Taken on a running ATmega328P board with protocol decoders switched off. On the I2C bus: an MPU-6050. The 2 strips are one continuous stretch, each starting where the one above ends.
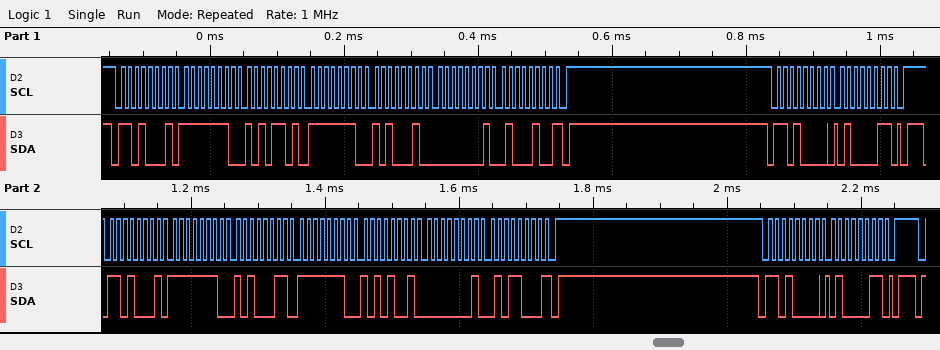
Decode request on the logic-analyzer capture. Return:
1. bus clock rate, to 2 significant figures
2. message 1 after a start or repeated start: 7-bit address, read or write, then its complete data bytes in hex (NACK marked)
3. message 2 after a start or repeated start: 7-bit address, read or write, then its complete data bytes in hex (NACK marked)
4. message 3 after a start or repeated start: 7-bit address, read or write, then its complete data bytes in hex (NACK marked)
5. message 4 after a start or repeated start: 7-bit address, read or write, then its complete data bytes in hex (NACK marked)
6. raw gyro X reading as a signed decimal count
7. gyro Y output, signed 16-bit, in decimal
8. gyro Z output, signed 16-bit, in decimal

100 kHz
0x68 read: FE AD FE A2 01 44 NACK
0x68 write: 43
0x68 read: FE A3 FE A9 01 58 NACK
0x68 write: 43
-349
-343
344
